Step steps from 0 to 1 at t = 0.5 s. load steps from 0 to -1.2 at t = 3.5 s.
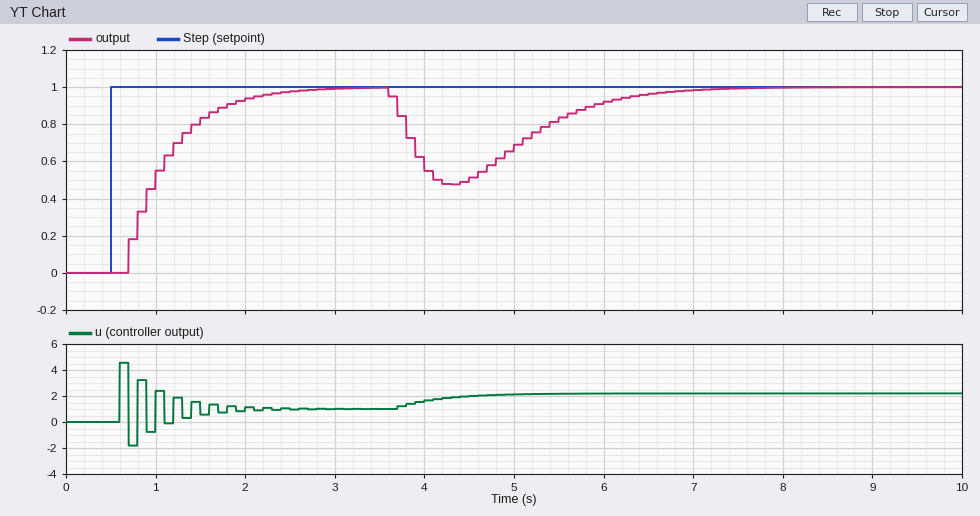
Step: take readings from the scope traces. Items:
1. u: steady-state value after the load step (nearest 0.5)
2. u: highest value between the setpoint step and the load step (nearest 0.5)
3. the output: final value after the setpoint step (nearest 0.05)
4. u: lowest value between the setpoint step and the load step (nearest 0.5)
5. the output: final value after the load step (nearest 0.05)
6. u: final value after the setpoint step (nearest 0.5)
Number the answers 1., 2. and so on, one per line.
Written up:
1. 2.0
2. 4.5
3. 1.00
4. -2.0
5. 1.00
6. 1.0
